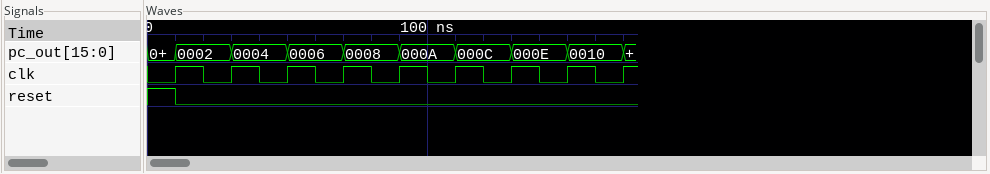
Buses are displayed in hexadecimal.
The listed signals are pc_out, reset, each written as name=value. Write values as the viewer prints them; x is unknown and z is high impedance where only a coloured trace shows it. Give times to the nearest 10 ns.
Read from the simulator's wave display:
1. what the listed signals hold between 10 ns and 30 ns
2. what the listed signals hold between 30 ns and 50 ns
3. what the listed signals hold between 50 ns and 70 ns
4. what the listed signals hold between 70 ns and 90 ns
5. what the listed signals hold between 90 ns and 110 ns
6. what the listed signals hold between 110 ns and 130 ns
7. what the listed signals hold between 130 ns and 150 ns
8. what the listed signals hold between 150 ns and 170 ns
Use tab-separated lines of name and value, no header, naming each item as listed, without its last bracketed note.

what the listed signals hold between 10 ns and 30 ns	pc_out=0002, reset=0
what the listed signals hold between 30 ns and 50 ns	pc_out=0004, reset=0
what the listed signals hold between 50 ns and 70 ns	pc_out=0006, reset=0
what the listed signals hold between 70 ns and 90 ns	pc_out=0008, reset=0
what the listed signals hold between 90 ns and 110 ns	pc_out=000A, reset=0
what the listed signals hold between 110 ns and 130 ns	pc_out=000C, reset=0
what the listed signals hold between 130 ns and 150 ns	pc_out=000E, reset=0
what the listed signals hold between 150 ns and 170 ns	pc_out=0010, reset=0
